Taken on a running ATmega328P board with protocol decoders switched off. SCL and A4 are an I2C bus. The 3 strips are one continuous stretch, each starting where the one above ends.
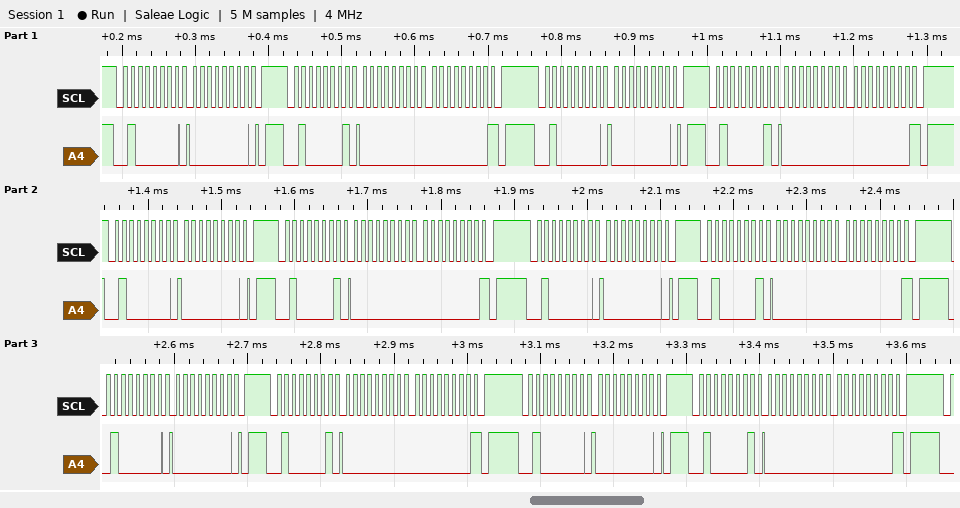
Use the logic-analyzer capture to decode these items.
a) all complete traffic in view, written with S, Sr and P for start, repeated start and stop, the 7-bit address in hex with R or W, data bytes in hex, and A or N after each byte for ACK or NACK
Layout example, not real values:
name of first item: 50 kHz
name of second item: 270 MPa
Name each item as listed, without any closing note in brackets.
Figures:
all complete traffic in view, written with S, Sr and P for start, repeated start and stop, the 7-bit address in hex with R or W, data bytes in hex, and A or N after each byte for ACK or NACK: S 20W A 00 A P S 20R A 00 A 00 N P S 20W A 00 A P S 20R A 00 A 00 N P S 20W A 00 A P S 20R A 00 A 00 N P S 20W A 00 A P S 20R A 00 A 00 N P S 20W A 00 A P S 20R A 00 A 00 N P S 20W A 00 A P S 20R A 00 A 00 N P
